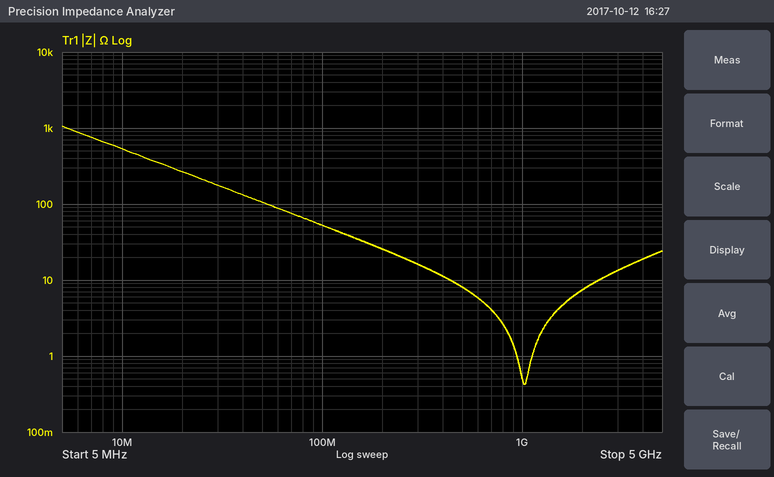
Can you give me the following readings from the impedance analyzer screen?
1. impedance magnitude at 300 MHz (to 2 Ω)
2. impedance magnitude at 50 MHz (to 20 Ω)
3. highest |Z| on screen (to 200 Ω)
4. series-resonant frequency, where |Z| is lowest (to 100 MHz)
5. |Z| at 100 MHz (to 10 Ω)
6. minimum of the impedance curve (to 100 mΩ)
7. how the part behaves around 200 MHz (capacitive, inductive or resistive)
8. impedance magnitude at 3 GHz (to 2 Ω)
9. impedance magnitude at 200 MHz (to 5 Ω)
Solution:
16 Ω
100 Ω
1.0 kΩ
1.0 GHz
50 Ω
400 mΩ
capacitive
14 Ω
25 Ω
